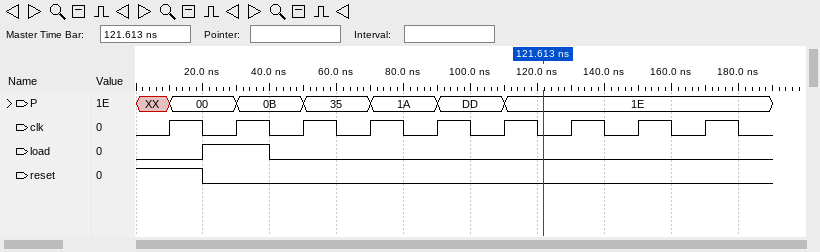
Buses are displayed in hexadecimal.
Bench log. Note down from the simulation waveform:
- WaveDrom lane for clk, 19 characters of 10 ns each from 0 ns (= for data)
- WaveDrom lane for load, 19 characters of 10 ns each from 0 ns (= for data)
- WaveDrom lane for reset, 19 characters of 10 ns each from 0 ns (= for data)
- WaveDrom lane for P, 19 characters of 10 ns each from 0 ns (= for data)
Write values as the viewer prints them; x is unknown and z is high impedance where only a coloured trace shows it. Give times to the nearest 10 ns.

{name: 'clk', wave: '0101010101010101010'}
{name: 'load', wave: '0.1.0..............'}
{name: 'reset', wave: '1.0................'}
{name: 'P', wave: 'x=.=.=.=.=.=.......', data: '00 0B 35 1A DD 1E'}
